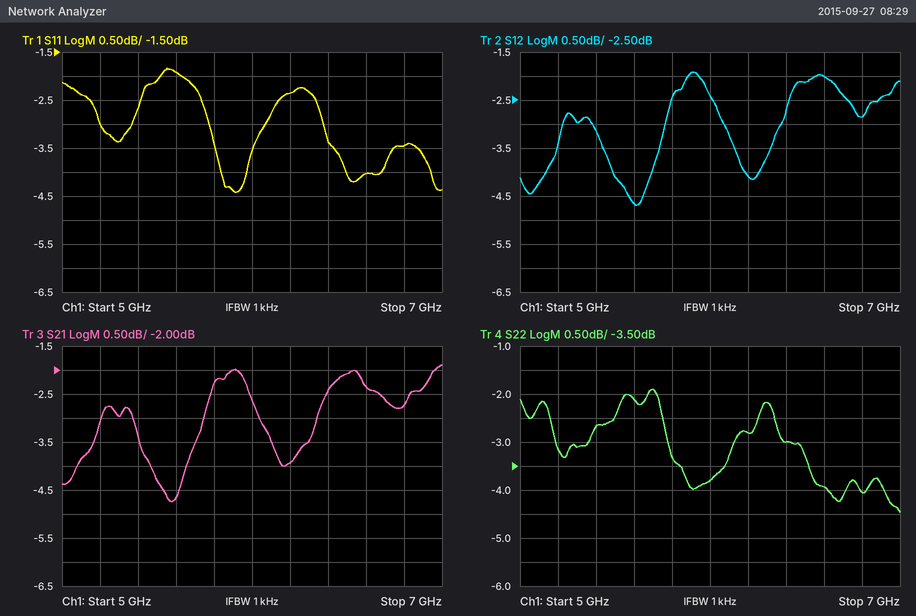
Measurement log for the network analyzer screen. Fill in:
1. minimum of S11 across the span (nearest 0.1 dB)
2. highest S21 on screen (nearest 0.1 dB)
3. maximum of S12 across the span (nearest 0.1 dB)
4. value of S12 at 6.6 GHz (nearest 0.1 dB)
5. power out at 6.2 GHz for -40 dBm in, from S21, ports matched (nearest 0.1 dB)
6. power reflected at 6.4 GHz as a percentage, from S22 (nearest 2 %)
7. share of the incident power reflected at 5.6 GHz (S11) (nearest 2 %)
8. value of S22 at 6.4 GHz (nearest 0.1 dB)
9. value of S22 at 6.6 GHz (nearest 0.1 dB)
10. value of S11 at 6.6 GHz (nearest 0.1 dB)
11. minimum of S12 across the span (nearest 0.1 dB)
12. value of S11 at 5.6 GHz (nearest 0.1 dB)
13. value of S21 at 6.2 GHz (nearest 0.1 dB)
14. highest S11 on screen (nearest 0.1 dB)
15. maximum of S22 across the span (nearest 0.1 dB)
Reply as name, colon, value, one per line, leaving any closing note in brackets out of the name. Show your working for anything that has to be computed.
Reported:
minimum of S11 across the span: -4.4 dB
highest S21 on screen: -1.9 dB
maximum of S12 across the span: -1.9 dB
value of S12 at 6.6 GHz: -2.0 dB
power out at 6.2 GHz for -40 dBm in, from S21, ports matched: -40 dBm + (-3.9 dB) = -43.9 dBm
power reflected at 6.4 GHz as a percentage, from S22: 10^(-3/10) ≈ 50 %
share of the incident power reflected at 5.6 GHz (S11): 10^(-1.9/10) ≈ 64.6 %, so 64 % to the nearest 2 %
value of S22 at 6.4 GHz: -3.0 dB
value of S22 at 6.6 GHz: -3.9 dB
value of S11 at 6.6 GHz: -4.0 dB
minimum of S12 across the span: -4.7 dB
value of S11 at 5.6 GHz: -1.9 dB
value of S21 at 6.2 GHz: -3.9 dB
highest S11 on screen: -1.8 dB
maximum of S22 across the span: -1.9 dB
